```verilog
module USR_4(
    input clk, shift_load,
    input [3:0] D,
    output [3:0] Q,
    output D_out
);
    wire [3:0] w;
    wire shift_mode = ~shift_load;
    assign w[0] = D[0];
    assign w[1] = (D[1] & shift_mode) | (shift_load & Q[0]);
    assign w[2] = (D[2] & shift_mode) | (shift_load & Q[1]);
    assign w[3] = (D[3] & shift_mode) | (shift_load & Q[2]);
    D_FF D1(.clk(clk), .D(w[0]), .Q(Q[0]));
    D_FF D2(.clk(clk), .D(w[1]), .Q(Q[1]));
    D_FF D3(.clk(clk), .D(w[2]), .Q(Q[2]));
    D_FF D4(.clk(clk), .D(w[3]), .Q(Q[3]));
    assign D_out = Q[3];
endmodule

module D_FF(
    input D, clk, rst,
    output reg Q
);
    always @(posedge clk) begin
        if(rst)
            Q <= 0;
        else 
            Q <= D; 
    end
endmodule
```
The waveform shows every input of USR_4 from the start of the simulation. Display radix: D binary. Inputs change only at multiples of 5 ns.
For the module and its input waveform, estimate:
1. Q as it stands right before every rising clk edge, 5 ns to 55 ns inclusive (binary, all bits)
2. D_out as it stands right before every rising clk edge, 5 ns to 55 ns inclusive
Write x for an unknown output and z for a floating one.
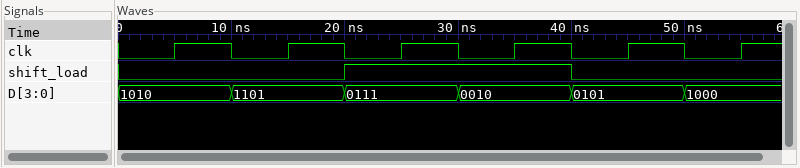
x, 1010, 1101, 1011, 0110, 0101
x 1 1 1 0 0
